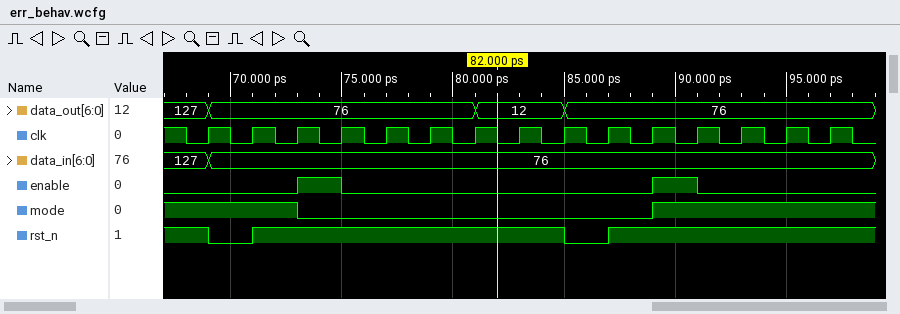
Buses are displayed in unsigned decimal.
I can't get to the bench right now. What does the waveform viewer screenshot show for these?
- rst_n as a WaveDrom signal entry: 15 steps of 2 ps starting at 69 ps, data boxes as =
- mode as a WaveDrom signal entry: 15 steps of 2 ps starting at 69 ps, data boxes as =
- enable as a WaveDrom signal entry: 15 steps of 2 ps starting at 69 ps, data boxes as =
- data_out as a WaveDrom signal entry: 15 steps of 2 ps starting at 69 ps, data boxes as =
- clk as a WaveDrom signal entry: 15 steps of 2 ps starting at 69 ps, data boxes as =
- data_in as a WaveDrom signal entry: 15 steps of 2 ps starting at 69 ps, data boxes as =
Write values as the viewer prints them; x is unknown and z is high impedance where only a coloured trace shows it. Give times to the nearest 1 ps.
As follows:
{name: 'rst_n', wave: '01......01.....'}
{name: 'mode', wave: '1.0.......1....'}
{name: 'enable', wave: '0.10......10...'}
{name: 'data_out', wave: '=.....=.=......', data: '76 12 76'}
{name: 'clk', wave: 'p..............'}
{name: 'data_in', wave: '=..............', data: '76'}
